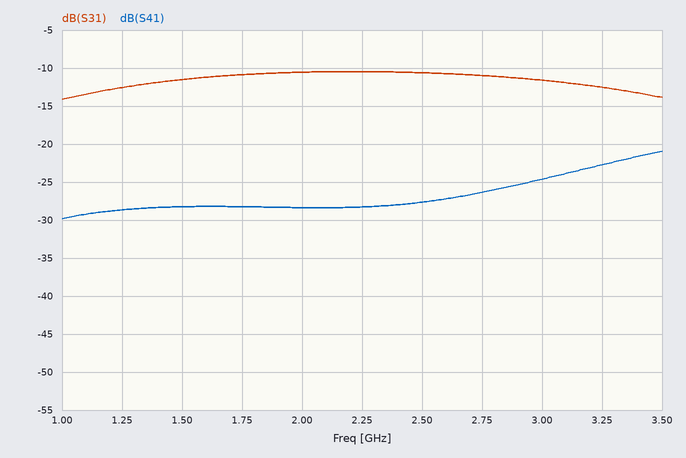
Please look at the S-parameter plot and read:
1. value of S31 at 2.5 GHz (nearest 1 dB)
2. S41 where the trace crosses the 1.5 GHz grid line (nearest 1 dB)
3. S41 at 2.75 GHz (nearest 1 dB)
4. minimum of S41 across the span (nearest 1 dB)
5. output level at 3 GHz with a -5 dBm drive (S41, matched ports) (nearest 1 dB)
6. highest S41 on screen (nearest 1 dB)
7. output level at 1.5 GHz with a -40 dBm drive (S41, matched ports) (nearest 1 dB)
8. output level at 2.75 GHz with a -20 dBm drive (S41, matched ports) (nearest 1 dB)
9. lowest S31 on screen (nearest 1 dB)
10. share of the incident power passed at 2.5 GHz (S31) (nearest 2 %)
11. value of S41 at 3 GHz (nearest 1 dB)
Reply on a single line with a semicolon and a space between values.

-11 dB; -28 dB; -26 dB; -30 dB; -30 dBm; -21 dB; -68 dBm; -46 dBm; -14 dB; 8 %; -25 dB
